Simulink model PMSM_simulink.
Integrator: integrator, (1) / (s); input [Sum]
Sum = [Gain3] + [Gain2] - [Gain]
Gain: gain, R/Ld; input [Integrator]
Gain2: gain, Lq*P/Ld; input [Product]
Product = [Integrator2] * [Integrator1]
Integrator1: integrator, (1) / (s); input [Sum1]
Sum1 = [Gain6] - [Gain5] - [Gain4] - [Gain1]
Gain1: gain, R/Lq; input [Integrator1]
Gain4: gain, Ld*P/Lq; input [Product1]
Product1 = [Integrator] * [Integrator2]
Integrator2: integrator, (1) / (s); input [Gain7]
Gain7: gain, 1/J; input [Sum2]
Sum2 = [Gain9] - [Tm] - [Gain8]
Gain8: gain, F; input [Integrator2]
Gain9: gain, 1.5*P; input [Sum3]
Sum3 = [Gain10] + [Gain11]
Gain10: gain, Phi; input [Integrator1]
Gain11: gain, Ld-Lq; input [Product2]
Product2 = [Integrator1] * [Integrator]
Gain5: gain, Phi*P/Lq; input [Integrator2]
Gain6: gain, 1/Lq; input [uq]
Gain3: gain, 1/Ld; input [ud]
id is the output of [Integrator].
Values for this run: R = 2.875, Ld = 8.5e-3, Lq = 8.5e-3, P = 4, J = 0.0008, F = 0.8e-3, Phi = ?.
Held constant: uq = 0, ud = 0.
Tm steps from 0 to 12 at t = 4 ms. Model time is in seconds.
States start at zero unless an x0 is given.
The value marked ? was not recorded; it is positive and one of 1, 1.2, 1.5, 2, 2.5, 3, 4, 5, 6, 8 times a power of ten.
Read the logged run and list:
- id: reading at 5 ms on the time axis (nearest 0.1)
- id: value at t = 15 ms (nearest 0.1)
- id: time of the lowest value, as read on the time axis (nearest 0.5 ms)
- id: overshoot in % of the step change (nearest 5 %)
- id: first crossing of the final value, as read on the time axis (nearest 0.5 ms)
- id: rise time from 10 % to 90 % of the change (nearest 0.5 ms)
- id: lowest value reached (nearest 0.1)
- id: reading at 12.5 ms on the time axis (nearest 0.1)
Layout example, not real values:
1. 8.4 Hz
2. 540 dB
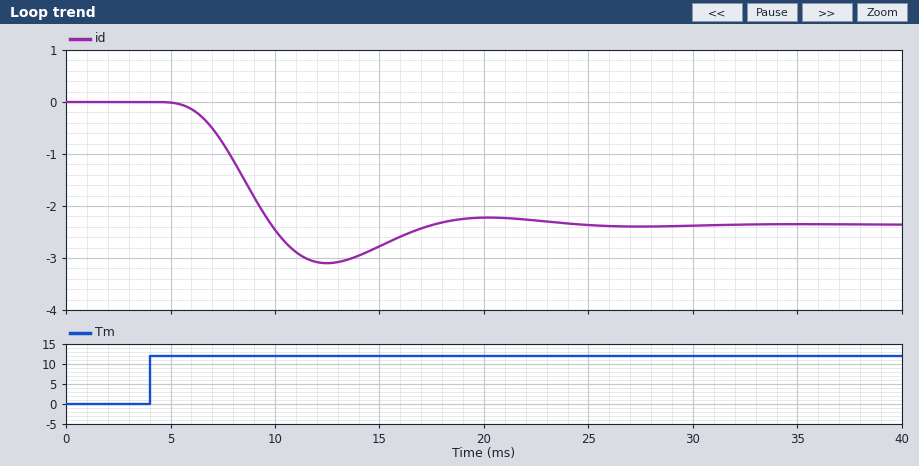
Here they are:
1. 0.0
2. -2.8
3. 12.5 ms
4. 30 %
5. 10.0 ms
6. 3.0 ms
7. -3.1
8. -3.1
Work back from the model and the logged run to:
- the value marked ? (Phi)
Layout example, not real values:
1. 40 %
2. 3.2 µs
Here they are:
1. 0.25
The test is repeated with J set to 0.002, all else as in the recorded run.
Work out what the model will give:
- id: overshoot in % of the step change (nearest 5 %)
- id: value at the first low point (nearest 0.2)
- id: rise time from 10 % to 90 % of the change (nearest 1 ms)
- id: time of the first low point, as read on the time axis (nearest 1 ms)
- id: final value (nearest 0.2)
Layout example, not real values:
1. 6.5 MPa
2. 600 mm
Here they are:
1. 10 %
2. -2.6
3. 7 ms
4. 20 ms
5. -2.4
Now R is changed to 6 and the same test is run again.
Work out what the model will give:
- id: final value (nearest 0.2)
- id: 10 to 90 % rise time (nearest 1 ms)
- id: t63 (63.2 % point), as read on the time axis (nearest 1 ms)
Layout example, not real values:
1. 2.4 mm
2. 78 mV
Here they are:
1. -2.4
2. 6 ms
3. 10 ms
